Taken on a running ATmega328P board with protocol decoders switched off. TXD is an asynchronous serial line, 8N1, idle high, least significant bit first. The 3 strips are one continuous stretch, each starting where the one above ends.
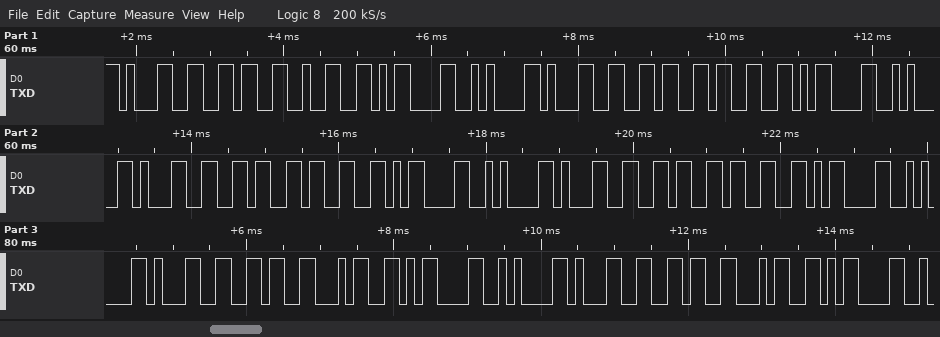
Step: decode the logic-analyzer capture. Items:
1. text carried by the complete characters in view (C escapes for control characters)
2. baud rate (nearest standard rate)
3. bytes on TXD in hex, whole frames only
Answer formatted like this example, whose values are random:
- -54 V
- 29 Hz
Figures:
- "162\r\n163\r\n163\r\n163\r\n164\r\n164\r"
- 9600 baud
- 31 36 32 0D 0A 31 36 33 0D 0A 31 36 33 0D 0A 31 36 33 0D 0A 31 36 34 0D 0A 31 36 34 0D
